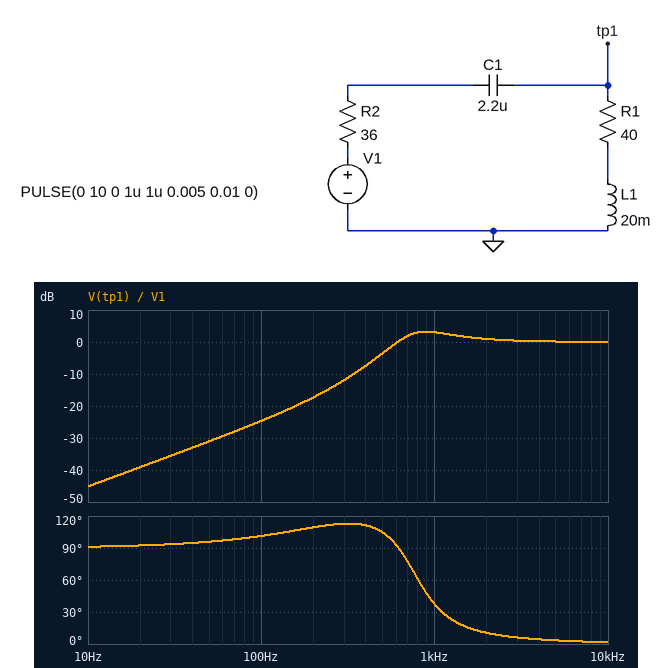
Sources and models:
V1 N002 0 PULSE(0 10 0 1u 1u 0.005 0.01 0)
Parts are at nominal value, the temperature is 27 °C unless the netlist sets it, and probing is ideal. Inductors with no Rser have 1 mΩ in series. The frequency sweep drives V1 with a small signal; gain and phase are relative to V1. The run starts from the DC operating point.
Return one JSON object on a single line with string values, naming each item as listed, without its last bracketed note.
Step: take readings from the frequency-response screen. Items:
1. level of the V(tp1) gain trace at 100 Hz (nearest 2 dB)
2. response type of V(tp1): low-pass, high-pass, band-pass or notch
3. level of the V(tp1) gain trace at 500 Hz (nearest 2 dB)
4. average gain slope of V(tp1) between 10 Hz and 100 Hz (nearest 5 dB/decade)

{"level of the V(tp1) gain trace at 100 Hz": "-24 dB", "response type of V(tp1): low-pass, high-pass, band-pass or notch": "high-pass", "level of the V(tp1) gain trace at 500 Hz": "-4 dB", "average gain slope of V(tp1) between 10 Hz and 100 Hz": "20 dB/decade"}
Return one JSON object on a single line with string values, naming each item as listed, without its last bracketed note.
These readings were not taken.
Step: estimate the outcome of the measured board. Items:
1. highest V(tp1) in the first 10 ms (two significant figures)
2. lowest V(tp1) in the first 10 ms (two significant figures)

{"highest V(tp1) in the first 10 ms": "10 V", "lowest V(tp1) in the first 10 ms": "-10 V"}
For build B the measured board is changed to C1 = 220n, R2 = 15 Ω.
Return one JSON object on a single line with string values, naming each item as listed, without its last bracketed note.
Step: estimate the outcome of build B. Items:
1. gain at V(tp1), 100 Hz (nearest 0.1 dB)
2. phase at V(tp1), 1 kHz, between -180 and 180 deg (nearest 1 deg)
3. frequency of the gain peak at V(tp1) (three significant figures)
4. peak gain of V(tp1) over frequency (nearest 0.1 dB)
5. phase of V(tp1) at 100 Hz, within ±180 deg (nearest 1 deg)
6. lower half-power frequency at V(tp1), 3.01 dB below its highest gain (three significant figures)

{"gain at V(tp1), 100 Hz": "-44.7 dB", "phase at V(tp1), 1 kHz, between -180 and 180 deg": "157 deg", "frequency of the gain peak at V(tp1)": "2.42 kHz", "peak gain of V(tp1) over frequency": "14.9 dB", "phase of V(tp1) at 100 Hz, within ±180 deg": "107 deg", "lower half-power frequency at V(tp1), 3.01 dB below its highest gain": "2.22 kHz"}
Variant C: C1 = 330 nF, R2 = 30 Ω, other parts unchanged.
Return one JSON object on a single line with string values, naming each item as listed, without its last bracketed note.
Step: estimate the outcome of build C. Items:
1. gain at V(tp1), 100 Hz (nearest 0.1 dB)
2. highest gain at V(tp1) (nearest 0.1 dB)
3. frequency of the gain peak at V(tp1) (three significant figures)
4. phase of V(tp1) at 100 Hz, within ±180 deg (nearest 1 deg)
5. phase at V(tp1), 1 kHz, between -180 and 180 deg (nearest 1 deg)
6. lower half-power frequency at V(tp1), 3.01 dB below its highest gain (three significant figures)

{"gain at V(tp1), 100 Hz": "-41.2 dB", "highest gain at V(tp1)": "11.1 dB", "frequency of the gain peak at V(tp1)": "2.00 kHz", "phase of V(tp1) at 100 Hz, within ±180 deg": "107 deg", "phase at V(tp1), 1 kHz, between -180 and 180 deg": "151 deg", "lower half-power frequency at V(tp1), 3.01 dB below its highest gain": "1.76 kHz"}
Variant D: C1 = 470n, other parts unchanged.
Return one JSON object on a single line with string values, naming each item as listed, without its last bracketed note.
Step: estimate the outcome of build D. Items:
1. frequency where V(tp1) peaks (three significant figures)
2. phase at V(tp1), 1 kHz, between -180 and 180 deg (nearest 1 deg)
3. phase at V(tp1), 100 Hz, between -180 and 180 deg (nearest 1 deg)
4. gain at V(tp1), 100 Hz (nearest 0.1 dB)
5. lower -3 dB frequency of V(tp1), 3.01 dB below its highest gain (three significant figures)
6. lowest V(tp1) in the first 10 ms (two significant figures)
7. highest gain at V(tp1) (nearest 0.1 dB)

{"frequency where V(tp1) peaks": "1.70 kHz", "phase at V(tp1), 1 kHz, between -180 and 180 deg": "143 deg", "phase at V(tp1), 100 Hz, between -180 and 180 deg": "106 deg", "gain at V(tp1), 100 Hz": "-38.1 dB", "lower -3 dB frequency of V(tp1), 3.01 dB below its highest gain": "1.44 kHz", "lowest V(tp1) in the first 10 ms": "-10 V", "highest gain at V(tp1)": "9.0 dB"}
